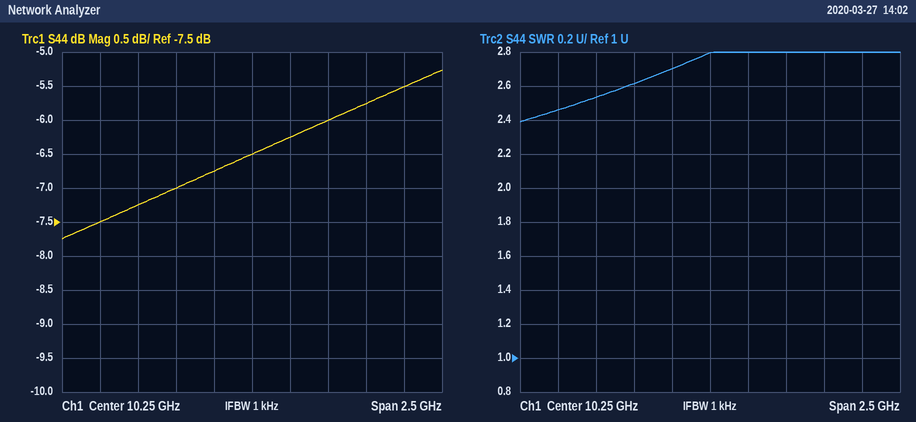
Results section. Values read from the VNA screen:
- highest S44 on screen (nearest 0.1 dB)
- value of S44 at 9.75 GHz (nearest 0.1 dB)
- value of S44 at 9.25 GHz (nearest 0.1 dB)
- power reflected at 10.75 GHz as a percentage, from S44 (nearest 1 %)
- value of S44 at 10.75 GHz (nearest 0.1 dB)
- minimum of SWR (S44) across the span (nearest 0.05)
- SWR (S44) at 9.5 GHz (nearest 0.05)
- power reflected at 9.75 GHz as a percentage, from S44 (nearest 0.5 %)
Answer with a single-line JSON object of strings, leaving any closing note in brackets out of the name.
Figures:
{"highest S44 on screen": "-5.3 dB", "value of S44 at 9.75 GHz": "-7.0 dB", "value of S44 at 9.25 GHz": "-7.5 dB", "power reflected at 10.75 GHz as a percentage, from S44": "25 %", "value of S44 at 10.75 GHz": "-6.0 dB", "minimum of SWR (S44) across the span": "2.40", "SWR (S44) at 9.5 GHz": "2.55", "power reflected at 9.75 GHz as a percentage, from S44": "20.0 %"}
